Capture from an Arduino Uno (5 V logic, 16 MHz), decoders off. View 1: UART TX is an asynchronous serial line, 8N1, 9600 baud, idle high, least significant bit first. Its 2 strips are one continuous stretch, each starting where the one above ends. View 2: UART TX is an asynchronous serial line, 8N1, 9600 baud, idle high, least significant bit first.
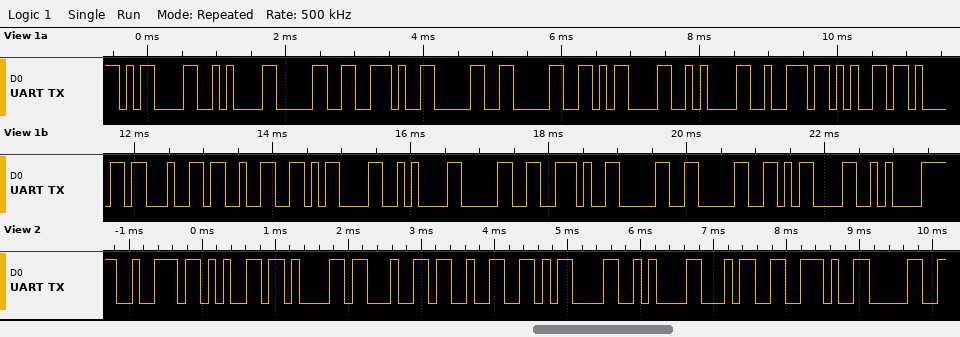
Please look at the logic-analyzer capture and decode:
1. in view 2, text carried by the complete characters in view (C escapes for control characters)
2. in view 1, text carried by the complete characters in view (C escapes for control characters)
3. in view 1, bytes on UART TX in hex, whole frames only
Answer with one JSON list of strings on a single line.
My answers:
["\"read2\\r\\n4.0\"", "\"\\r\\n0.00\\r\\nread2\\r\\n0.00\\r\\n\"", "0D 0A 30 2E 30 30 0D 0A 72 65 61 64 32 0D 0A 30 2E 30 30 0D 0A"]
